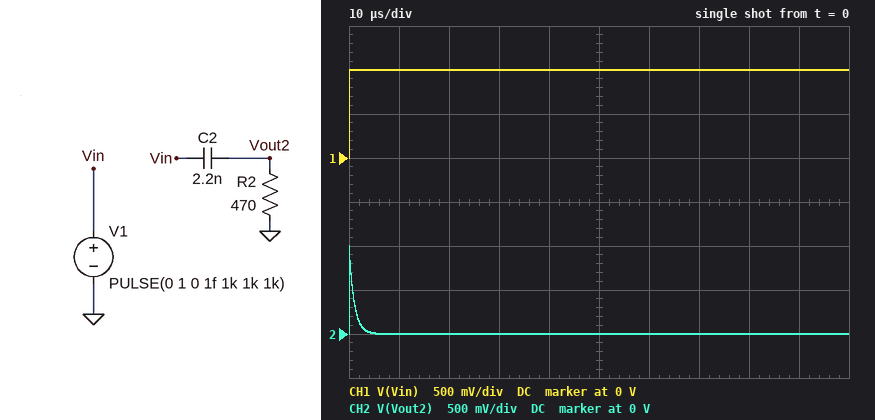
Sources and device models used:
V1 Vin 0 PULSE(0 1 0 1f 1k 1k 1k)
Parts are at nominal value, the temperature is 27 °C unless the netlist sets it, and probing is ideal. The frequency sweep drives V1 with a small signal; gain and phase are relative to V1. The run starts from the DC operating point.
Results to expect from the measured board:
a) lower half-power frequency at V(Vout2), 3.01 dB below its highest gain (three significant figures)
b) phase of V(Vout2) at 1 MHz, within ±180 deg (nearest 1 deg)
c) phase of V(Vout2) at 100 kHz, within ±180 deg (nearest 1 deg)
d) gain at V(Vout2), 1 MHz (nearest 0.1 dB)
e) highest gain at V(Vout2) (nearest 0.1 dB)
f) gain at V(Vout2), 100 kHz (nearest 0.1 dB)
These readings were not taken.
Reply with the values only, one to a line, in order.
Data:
154 kHz
9 deg
57 deg
-0.1 dB
0 dB
-5.3 dB
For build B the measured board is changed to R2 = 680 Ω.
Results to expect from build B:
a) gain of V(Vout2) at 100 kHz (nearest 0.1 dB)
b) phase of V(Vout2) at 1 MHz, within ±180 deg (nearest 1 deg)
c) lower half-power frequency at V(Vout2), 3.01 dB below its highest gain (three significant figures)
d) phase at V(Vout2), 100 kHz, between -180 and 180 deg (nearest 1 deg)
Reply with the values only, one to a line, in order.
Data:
-3.3 dB
6 deg
106 kHz
47 deg
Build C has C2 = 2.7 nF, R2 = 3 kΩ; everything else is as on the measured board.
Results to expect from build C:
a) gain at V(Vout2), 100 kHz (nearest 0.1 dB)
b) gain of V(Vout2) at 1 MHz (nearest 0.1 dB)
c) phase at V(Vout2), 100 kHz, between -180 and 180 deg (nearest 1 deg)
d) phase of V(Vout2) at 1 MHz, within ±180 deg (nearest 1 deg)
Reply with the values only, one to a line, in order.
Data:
-0.2 dB
0 dB
11 deg
1 deg
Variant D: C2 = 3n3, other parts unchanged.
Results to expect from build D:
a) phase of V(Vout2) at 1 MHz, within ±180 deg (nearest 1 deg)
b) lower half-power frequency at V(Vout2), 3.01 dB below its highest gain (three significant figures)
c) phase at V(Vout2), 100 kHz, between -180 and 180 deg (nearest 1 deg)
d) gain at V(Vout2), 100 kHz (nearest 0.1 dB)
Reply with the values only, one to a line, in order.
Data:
6 deg
103 kHz
46 deg
-3.1 dB
